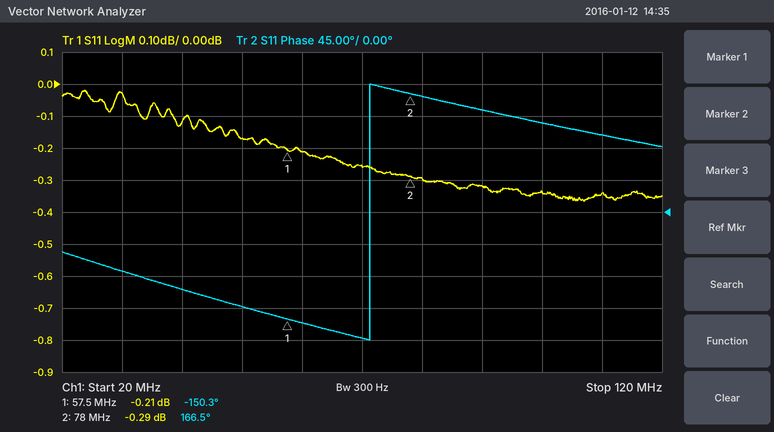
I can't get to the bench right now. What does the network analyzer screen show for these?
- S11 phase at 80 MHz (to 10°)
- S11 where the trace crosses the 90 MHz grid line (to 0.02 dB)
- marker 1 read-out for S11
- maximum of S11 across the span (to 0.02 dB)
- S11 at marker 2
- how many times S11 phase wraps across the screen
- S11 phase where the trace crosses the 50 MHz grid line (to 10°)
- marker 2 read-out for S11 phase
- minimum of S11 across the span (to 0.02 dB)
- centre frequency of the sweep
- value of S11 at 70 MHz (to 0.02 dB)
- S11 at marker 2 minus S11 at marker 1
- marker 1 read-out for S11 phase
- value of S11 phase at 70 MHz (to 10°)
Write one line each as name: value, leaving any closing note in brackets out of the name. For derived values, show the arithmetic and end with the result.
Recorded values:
S11 phase at 80 MHz: 160°
S11 where the trace crosses the 90 MHz grid line: -0.32 dB
marker 1 read-out for S11: -0.21 dB
maximum of S11 across the span: -0.02 dB
S11 at marker 2: -0.29 dB
how many times S11 phase wraps across the screen: 1
S11 phase where the trace crosses the 50 MHz grid line: -130°
marker 2 read-out for S11 phase: 166.5°
minimum of S11 across the span: -0.36 dB
centre frequency of the sweep: 70 MHz
value of S11 at 70 MHz: -0.26 dB
S11 at marker 2 minus S11 at marker 1: -0.29 − (-0.21) = -0.08 dB
marker 1 read-out for S11 phase: -150.3°
value of S11 phase at 70 MHz: -180°
